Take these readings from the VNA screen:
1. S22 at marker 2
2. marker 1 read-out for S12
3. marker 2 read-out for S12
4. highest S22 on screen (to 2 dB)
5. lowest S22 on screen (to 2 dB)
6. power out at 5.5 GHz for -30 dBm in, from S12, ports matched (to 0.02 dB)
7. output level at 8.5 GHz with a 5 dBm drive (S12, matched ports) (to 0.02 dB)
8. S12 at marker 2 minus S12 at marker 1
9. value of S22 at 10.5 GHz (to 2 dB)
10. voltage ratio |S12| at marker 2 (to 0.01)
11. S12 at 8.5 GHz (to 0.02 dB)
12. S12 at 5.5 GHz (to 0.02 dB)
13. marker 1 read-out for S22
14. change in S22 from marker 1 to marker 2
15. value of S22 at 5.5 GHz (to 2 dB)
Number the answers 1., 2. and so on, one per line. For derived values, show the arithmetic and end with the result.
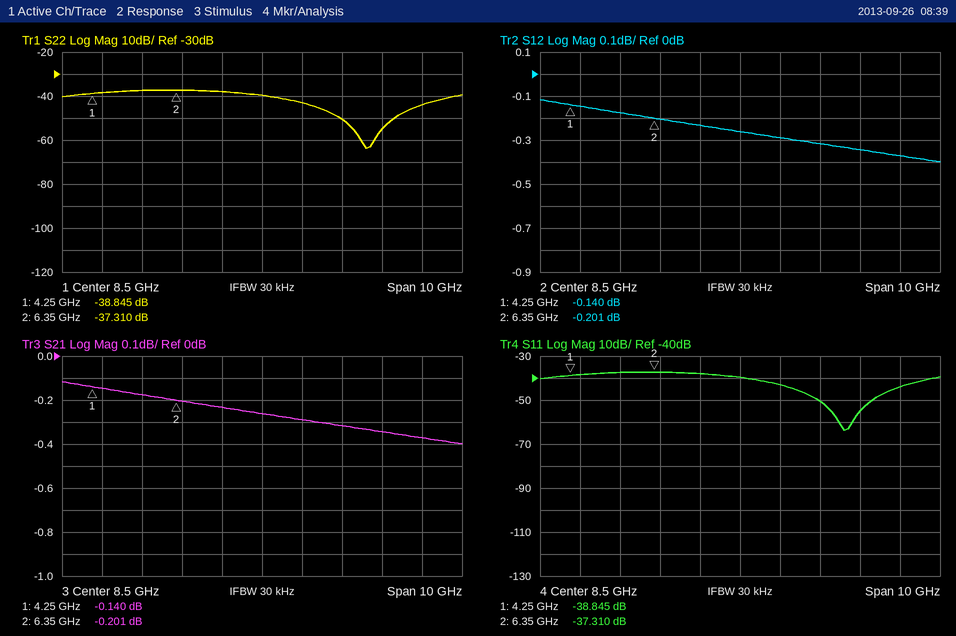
1. -37.310 dB
2. -0.140 dB
3. -0.201 dB
4. -38 dB
5. -64 dB
6. -30 dBm + (-0.18 dB) = -30.18 dBm
7. 5 dBm + (-0.26 dB) = 4.74 dBm
8. -0.201 − (-0.14) = -0.061 dB
9. -50 dB
10. 10^(-0.201/20) ≈ 0.98
11. -0.26 dB
12. -0.18 dB
13. -38.845 dB
14. -37.31 − (-38.845) = 1.535 dB
15. -38 dB
